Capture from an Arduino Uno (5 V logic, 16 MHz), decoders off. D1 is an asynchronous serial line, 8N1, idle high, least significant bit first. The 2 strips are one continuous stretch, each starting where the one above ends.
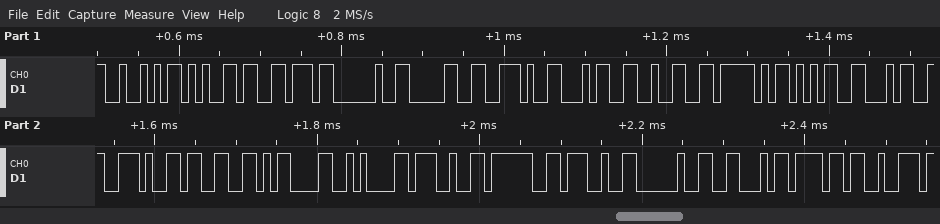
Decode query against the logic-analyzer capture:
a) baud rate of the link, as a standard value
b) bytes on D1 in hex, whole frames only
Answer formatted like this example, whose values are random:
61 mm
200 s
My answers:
115200 baud
52 65 76 20 30 2E 34 32 5F 35 34 2E 33 0D 0A 27 3F 27 20 46 6F 72
